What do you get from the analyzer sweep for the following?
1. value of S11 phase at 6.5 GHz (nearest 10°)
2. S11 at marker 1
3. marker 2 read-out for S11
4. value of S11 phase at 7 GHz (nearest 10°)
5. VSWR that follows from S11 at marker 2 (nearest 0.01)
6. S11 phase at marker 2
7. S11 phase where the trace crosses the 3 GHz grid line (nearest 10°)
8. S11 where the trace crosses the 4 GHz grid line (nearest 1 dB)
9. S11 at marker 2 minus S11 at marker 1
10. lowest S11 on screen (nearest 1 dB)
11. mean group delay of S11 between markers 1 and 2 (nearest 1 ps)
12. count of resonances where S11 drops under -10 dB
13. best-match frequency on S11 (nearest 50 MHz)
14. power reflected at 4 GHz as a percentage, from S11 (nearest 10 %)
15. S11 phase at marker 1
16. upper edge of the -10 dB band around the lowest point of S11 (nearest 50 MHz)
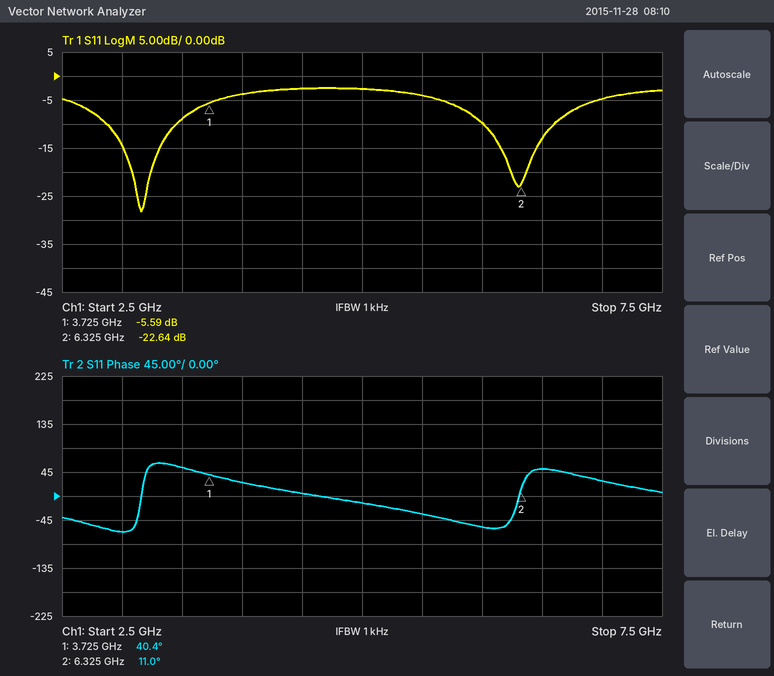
50°
-5.59 dB
-22.64 dB
30°
1.16
11.0°
-70°
-4 dB
-17.05 dB
-28 dB
31 ps
2
3.15 GHz
40 %
40.4°
3.45 GHz
